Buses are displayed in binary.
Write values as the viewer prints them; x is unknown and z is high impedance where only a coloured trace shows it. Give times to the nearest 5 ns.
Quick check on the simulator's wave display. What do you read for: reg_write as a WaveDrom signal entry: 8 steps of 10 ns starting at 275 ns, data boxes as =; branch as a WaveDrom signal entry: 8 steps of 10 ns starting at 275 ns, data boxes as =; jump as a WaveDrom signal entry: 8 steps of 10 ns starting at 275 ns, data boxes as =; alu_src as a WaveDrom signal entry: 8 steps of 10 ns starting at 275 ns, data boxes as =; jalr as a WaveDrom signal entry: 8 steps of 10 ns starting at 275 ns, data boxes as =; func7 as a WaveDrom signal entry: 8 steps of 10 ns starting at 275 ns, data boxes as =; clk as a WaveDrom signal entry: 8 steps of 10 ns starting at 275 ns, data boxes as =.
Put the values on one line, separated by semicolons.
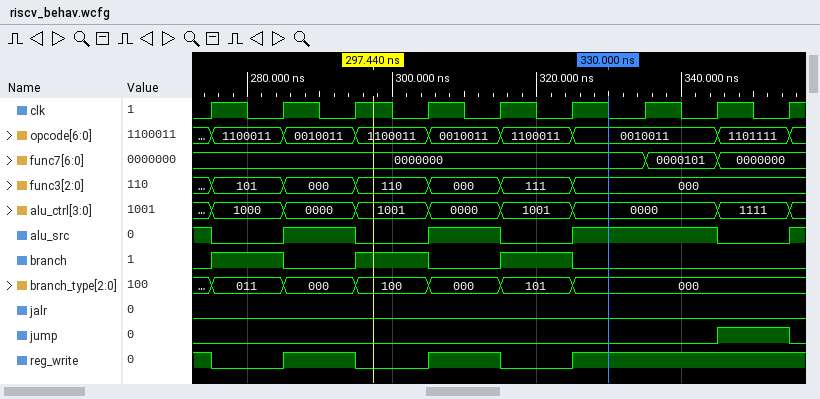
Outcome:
{name: 'reg_write', wave: '010101..'}; {name: 'branch', wave: '101010..'}; {name: 'jump', wave: '0......1'}; {name: 'alu_src', wave: '010101.0'}; {name: 'jalr', wave: '0.......'}; {name: 'func7', wave: '=.....==', data: '0000000 0000101 0000000'}; {name: 'clk', wave: 'p.......'}
